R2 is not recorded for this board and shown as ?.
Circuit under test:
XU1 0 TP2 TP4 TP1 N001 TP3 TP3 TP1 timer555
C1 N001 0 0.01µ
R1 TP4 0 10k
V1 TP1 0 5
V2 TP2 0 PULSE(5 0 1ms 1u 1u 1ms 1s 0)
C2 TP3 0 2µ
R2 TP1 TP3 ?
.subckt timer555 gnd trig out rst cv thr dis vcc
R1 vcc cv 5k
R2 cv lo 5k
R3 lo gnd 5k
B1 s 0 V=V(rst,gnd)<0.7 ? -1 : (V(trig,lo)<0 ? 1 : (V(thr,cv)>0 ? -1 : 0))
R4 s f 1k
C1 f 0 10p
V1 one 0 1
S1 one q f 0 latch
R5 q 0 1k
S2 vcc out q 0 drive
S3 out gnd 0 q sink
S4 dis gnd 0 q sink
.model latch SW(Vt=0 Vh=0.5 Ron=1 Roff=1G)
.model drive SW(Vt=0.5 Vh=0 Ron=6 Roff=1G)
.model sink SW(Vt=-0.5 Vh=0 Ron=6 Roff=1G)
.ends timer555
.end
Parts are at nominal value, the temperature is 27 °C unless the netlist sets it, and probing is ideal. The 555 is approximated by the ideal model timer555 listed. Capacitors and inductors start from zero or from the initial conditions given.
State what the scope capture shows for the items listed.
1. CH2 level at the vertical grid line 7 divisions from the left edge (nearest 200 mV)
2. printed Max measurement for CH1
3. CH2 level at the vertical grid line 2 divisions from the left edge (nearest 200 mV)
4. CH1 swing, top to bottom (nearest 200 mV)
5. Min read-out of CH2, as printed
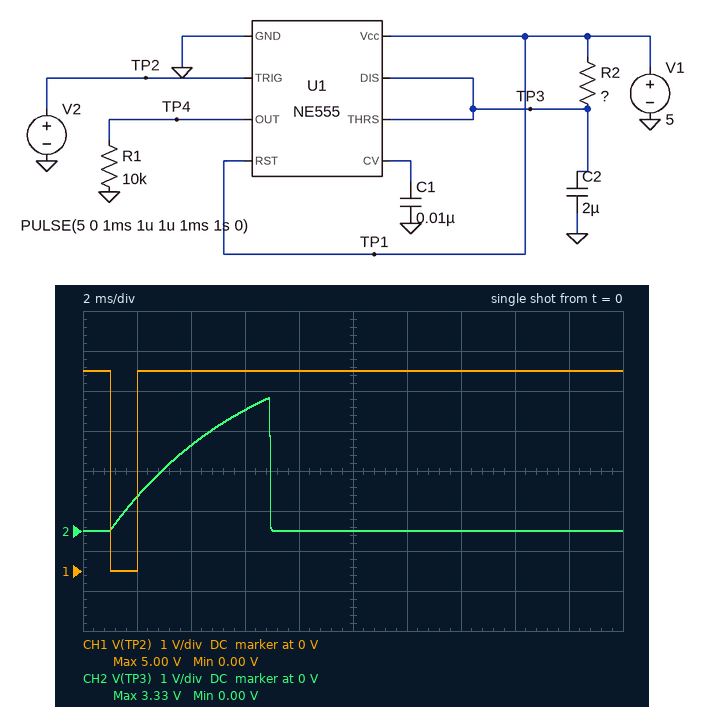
0 V
5.00 V
2.2 V
5.0 V
0.00 V
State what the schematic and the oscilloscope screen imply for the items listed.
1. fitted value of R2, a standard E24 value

2.7 kΩ
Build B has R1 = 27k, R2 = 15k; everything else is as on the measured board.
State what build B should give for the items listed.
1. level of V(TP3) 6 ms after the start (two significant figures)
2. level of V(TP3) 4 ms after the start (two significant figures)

770 mV
480 mV
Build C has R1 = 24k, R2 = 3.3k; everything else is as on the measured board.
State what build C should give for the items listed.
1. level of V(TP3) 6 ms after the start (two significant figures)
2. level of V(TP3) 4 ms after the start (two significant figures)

2.7 V
1.8 V
